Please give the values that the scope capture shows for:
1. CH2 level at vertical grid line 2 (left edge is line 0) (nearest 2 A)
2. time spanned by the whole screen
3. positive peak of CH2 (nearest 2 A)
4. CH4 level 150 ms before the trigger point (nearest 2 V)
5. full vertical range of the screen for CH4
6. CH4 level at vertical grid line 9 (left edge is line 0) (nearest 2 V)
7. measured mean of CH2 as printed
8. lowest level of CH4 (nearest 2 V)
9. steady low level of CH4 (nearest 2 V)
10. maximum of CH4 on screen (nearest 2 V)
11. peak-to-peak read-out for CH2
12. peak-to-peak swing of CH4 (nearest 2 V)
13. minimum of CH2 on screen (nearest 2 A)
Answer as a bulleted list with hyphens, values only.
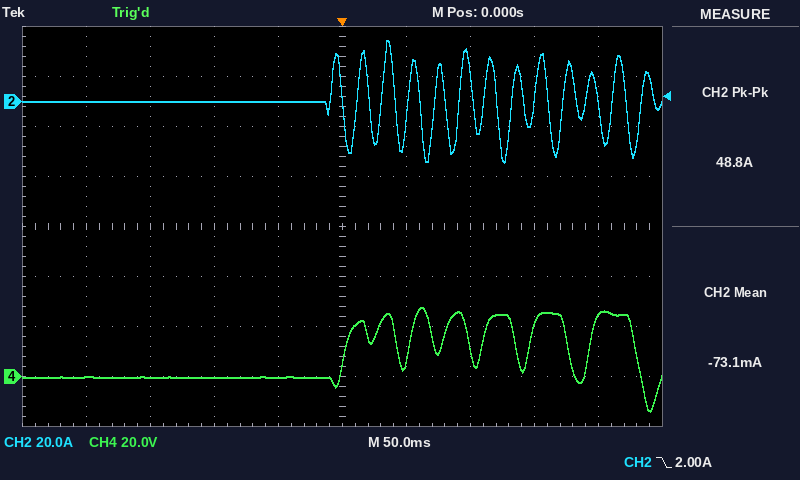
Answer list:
- 0 A
- 500 ms
- 24 A
- 0 V
- 160 V
- 24 V
- -73.1 mA
- -14 V
- 0 V
- 28 V
- 48.8 A
- 42 V
- -24 A
